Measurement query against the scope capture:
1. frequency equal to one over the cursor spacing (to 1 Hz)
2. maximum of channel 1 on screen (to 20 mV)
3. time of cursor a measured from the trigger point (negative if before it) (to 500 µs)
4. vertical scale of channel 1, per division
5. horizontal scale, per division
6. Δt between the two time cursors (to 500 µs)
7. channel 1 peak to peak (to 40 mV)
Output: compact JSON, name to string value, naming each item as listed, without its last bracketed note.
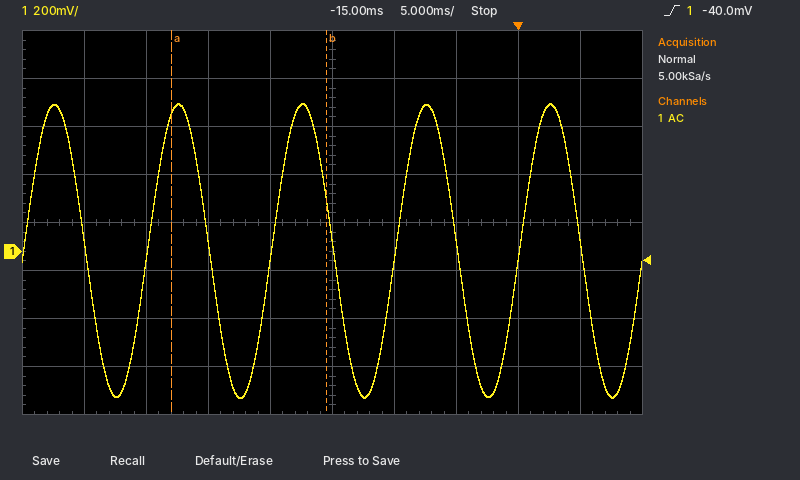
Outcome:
{"frequency equal to one over the cursor spacing": "80 Hz", "maximum of channel 1 on screen": "620 mV", "time of cursor a measured from the trigger point (negative if before it)": "-28.0 ms", "vertical scale of channel 1, per division": "200 mV", "horizontal scale, per division": "5 ms", "Δt between the two time cursors": "12.5 ms", "channel 1 peak to peak": "1.24 V"}
